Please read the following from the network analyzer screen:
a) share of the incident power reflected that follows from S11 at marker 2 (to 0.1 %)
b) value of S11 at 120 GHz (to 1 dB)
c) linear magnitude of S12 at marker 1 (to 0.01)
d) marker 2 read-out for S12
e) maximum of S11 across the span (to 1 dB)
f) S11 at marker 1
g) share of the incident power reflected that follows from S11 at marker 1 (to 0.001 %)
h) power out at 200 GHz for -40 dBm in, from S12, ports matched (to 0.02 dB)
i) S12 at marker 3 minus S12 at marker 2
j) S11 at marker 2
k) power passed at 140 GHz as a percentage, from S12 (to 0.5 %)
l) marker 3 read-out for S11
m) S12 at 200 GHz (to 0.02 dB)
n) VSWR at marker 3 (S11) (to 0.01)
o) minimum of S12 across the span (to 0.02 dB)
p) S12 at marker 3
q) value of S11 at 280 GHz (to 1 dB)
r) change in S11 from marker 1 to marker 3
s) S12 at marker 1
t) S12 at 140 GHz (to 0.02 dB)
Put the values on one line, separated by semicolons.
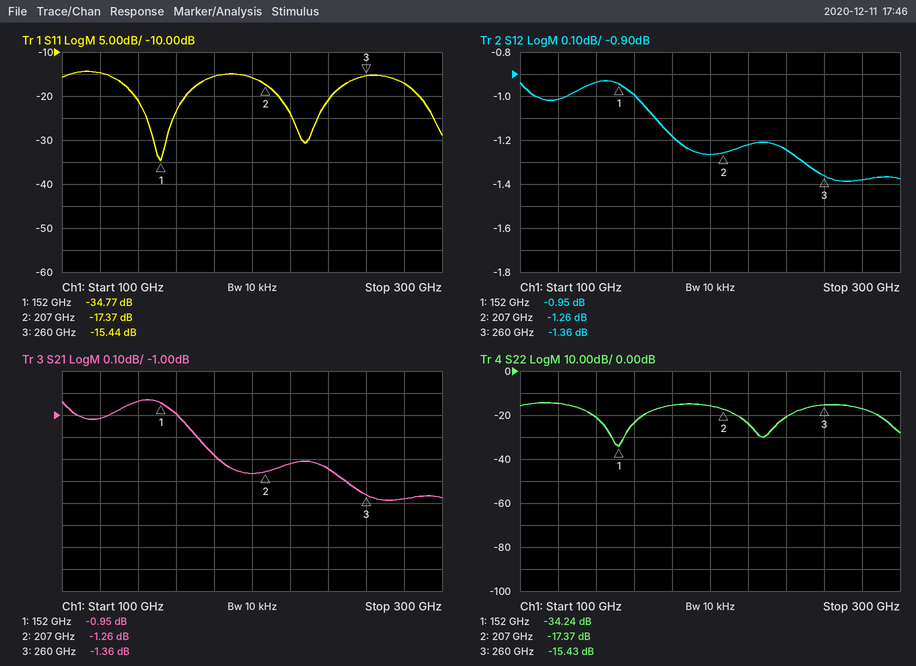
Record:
1.8 %; -15 dB; 0.90; -1.26 dB; -14 dB; -34.77 dB; 0.033 %; -41.26 dBm; -0.10 dB; -17.37 dB; 80.5 %; -15.44 dB; -1.26 dB; 1.41; -1.38 dB; -1.36 dB; -17 dB; 19.33 dB; -0.95 dB; -0.94 dB
